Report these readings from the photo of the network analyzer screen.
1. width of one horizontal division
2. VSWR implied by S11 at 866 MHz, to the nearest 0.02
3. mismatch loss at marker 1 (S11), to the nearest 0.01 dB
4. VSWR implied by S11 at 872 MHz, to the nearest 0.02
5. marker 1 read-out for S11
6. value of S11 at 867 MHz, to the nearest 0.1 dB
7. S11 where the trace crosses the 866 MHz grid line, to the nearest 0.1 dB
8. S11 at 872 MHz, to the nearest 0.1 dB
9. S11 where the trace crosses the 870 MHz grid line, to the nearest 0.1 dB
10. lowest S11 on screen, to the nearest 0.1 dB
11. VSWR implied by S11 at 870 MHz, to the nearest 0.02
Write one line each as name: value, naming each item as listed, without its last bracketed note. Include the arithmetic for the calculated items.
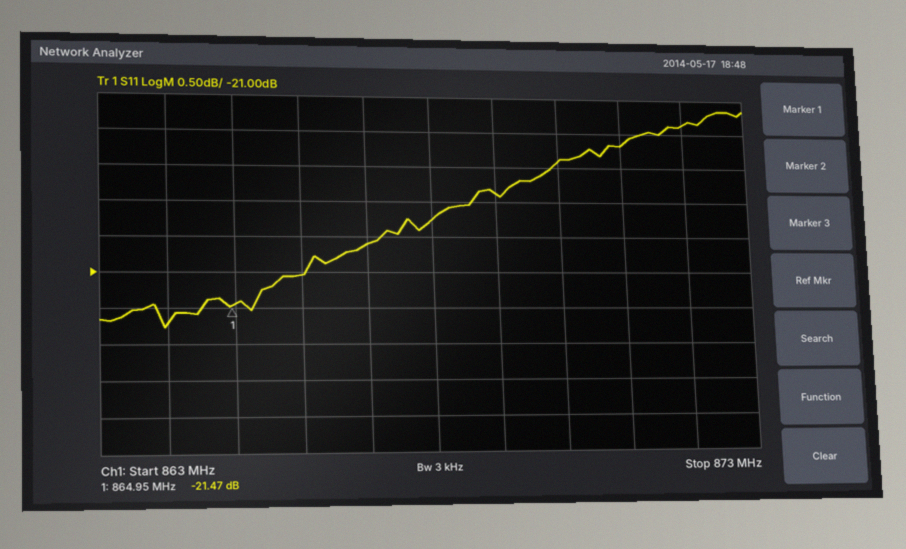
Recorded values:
width of one horizontal division: 1 MHz
VSWR implied by S11 at 866 MHz, to the nearest 0.02: |Γ| = 10^(-21/20) = 0.0891; VSWR = (1 + 0.0891)/(1 − 0.0891) ≈ 1.20
mismatch loss at marker 1 (S11), to the nearest 0.01 dB: −10 log10(1 − 10^(-21.47/10)) ≈ 0.03 dB
VSWR implied by S11 at 872 MHz, to the nearest 0.02: |Γ| = 10^(-18.9/20) = 0.1135; VSWR = (1 + 0.1135)/(1 − 0.1135) ≈ 1.26
marker 1 read-out for S11: -21.47 dB
value of S11 at 867 MHz, to the nearest 0.1 dB: -20.6 dB
S11 where the trace crosses the 866 MHz grid line, to the nearest 0.1 dB: -21.0 dB
S11 at 872 MHz, to the nearest 0.1 dB: -18.9 dB
S11 where the trace crosses the 870 MHz grid line, to the nearest 0.1 dB: -19.4 dB
lowest S11 on screen, to the nearest 0.1 dB: -21.8 dB
VSWR implied by S11 at 870 MHz, to the nearest 0.02: |Γ| = 10^(-19.4/20) = 0.1072; VSWR = (1 + 0.1072)/(1 − 0.1072) ≈ 1.24
